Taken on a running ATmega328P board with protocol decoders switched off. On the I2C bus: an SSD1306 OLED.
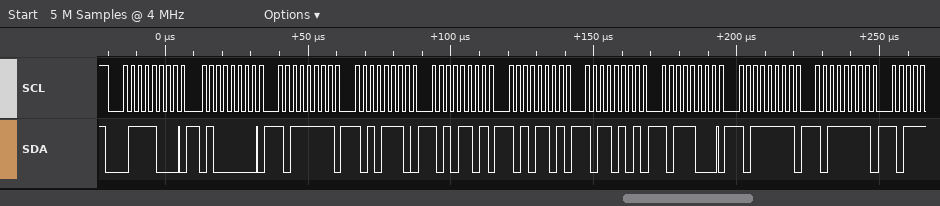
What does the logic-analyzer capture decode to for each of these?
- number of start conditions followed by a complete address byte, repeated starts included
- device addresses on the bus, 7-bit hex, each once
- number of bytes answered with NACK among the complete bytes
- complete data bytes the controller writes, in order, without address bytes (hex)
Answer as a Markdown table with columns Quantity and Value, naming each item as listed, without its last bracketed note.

| Quantity | Value |
|---|---|
| number of start conditions followed by a complete address byte, repeated starts included | 1 |
| device addresses on the bus, 7-bit hex, each once | 0x3C |
| number of bytes answered with NACK among the complete bytes | 0 |
| complete data bytes the controller writes, in order, without address bytes | 40 BF AE AD AD B5 B8 BF BF |
